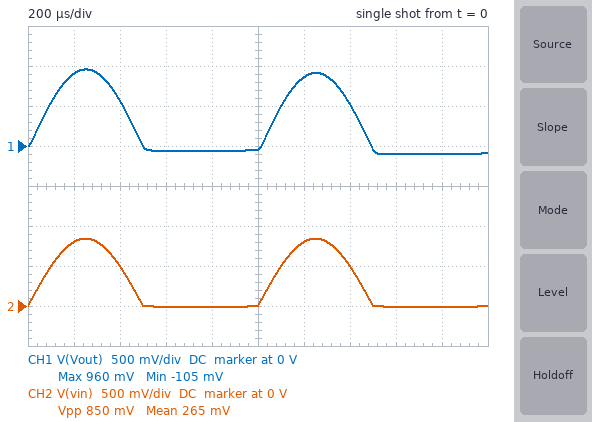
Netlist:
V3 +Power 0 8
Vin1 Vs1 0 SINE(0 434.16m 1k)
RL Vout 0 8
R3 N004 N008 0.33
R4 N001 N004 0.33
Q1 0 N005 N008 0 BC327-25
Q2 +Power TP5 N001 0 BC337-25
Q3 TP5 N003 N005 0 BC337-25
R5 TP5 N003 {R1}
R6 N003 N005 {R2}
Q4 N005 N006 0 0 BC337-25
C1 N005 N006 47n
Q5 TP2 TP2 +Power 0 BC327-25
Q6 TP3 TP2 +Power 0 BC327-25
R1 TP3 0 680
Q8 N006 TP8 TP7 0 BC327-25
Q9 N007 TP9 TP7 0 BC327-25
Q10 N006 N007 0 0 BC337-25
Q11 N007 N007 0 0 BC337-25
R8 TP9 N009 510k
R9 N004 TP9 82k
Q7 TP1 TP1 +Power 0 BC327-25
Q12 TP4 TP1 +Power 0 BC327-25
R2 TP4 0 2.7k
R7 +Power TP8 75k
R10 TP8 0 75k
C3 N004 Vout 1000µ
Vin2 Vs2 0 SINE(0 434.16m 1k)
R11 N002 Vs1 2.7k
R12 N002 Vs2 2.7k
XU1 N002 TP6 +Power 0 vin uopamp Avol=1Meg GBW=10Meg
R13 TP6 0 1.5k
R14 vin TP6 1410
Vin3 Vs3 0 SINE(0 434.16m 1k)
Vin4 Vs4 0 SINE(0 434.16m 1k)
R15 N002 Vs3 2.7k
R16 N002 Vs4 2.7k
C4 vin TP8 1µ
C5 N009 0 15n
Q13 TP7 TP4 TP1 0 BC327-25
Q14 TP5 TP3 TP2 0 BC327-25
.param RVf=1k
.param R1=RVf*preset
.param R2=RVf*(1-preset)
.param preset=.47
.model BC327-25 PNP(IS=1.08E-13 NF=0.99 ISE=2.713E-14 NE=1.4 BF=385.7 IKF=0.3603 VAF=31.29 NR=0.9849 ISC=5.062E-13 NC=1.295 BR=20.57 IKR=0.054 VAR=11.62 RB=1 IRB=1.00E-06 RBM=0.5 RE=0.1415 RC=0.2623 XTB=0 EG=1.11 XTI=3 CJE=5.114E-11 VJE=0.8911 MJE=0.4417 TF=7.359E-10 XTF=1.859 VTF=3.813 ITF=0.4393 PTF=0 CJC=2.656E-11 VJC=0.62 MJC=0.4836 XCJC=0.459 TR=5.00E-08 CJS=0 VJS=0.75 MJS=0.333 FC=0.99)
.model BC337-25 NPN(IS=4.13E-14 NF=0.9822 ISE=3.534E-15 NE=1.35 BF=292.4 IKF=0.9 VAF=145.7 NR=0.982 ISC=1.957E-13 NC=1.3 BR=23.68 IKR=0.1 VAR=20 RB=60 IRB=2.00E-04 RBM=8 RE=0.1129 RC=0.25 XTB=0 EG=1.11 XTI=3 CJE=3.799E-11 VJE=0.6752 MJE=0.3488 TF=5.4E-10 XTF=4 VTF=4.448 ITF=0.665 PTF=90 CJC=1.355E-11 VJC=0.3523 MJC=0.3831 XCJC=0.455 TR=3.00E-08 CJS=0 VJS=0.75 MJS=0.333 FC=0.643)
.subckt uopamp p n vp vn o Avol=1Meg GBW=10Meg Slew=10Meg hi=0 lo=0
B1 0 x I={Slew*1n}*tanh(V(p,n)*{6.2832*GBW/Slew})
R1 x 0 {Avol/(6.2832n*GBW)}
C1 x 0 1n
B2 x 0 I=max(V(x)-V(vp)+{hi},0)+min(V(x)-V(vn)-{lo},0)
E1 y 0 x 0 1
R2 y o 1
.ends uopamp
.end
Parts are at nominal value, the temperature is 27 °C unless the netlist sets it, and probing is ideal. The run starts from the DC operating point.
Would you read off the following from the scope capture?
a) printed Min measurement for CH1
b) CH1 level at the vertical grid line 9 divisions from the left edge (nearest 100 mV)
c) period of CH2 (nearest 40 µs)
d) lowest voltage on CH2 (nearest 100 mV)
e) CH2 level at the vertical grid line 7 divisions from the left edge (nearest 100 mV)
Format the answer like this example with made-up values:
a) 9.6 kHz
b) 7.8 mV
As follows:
a) -105 mV
b) -100 mV
c) 1.00 ms
d) 0 V
e) 500 mV
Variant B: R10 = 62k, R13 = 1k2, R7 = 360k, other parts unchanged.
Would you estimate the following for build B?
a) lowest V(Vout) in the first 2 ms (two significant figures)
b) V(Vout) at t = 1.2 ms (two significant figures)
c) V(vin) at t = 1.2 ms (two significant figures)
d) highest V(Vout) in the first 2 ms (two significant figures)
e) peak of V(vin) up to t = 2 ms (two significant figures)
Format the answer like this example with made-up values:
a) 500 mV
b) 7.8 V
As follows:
a) -110 mV
b) 970 mV
c) 900 mV
d) 1.1 V
e) 940 mV
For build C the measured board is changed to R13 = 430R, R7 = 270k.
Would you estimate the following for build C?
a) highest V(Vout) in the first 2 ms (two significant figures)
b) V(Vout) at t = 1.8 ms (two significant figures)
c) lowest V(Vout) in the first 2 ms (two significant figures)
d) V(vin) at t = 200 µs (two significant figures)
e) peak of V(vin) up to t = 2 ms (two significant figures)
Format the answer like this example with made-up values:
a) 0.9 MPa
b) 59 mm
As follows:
a) 2.1 V
b) -200 mV
c) -210 mV
d) 1.8 V
e) 1.9 V
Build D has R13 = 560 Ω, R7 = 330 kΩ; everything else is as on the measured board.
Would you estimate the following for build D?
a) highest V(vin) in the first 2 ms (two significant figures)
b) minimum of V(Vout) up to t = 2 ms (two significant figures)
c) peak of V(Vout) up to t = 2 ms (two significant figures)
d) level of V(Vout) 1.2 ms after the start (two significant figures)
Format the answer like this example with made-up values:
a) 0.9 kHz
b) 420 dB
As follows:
a) 1.5 V
b) -170 mV
c) 1.7 V
d) 1.6 V
